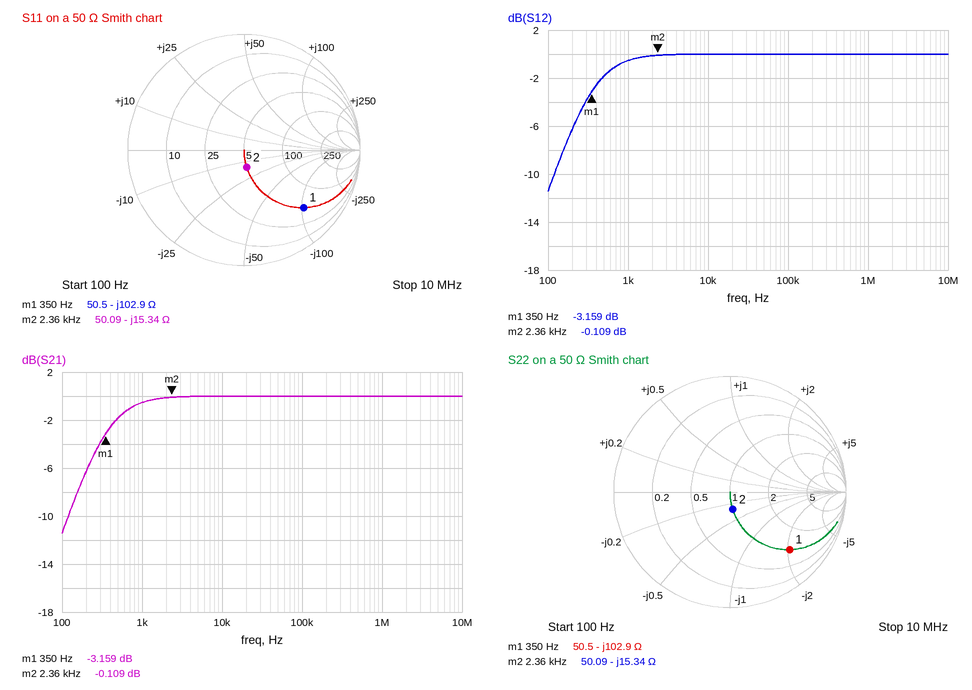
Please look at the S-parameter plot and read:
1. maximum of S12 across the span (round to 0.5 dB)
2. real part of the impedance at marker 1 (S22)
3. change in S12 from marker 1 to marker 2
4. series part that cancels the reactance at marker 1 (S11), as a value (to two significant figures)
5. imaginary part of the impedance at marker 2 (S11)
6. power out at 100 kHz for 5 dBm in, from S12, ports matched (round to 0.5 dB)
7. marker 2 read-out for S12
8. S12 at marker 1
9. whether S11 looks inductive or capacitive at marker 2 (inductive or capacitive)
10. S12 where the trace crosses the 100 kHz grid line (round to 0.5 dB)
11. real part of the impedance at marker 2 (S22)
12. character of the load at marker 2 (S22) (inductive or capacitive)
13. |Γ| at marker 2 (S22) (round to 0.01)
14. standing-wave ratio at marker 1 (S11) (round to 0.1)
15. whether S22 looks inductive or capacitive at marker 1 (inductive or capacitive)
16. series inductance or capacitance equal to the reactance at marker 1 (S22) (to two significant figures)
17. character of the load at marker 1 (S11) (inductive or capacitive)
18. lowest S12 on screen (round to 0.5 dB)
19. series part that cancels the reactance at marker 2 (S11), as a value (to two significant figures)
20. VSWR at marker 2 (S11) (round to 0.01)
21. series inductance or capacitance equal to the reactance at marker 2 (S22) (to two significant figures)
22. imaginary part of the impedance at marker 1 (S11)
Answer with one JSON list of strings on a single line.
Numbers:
["0.0 dB", "50.5 Ω", "3.050 dB", "47 mH", "-15.34 Ω", "5.0 dBm", "-0.109 dB", "-3.159 dB", "capacitive", "0.0 dB", "50.09 Ω", "capacitive", "0.15", "6.0", "capacitive", "4.4 µF", "capacitive", "-11.5 dB", "1.0 mH", "1.36", "4.4 µF", "-102.9 Ω"]
